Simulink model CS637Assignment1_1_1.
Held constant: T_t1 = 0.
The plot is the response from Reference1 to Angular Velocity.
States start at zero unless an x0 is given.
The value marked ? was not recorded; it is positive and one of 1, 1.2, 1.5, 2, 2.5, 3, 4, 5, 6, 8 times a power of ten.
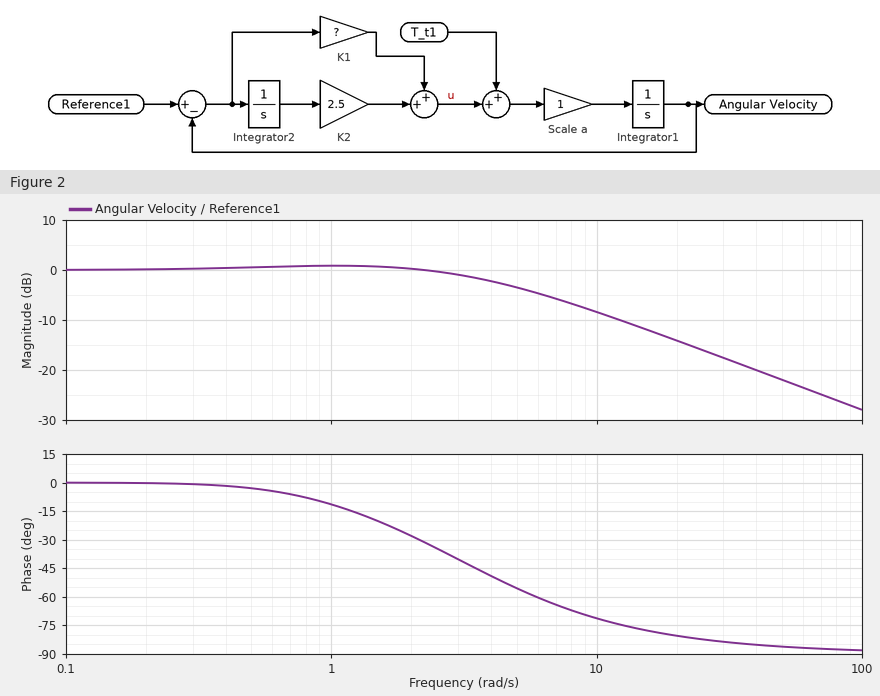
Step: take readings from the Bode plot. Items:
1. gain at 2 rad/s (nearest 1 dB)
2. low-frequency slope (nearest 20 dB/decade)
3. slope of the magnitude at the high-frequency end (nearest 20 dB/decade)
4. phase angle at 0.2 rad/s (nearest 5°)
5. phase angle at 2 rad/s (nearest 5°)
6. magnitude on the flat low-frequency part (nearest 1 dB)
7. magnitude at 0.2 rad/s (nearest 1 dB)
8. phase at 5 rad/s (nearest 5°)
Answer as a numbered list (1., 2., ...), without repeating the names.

1. 0 dB
2. 0 dB/decade
3. -20 dB/decade
4. 0°
5. -30°
6. 0 dB
7. 0 dB
8. -55°
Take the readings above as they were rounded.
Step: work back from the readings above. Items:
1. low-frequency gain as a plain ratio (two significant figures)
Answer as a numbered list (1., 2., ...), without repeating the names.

1. 1.0
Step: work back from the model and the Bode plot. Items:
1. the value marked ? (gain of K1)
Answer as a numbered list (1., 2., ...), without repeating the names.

1. 4
